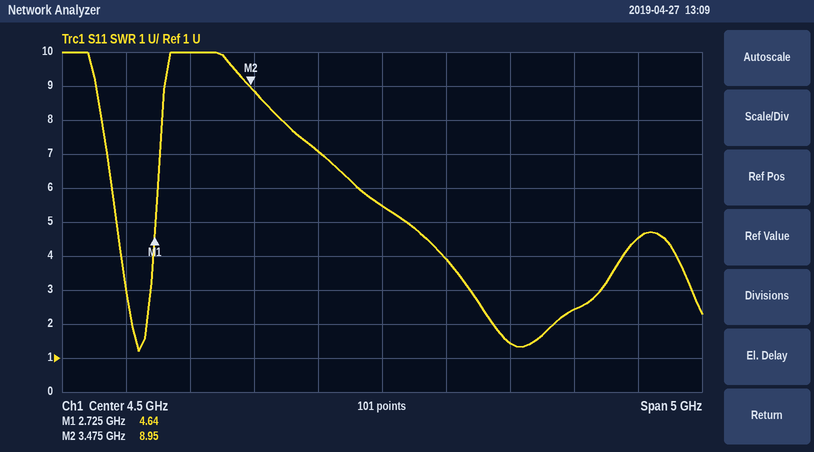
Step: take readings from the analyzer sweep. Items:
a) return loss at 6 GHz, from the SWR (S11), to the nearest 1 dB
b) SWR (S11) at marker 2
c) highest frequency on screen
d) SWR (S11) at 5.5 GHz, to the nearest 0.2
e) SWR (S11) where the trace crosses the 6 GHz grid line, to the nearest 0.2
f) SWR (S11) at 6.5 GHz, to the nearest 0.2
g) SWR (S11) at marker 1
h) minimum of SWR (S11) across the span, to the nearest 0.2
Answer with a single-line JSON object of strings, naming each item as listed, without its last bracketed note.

{"return loss at 6 GHz, from the SWR (S11), to the nearest 1 dB": "8 dB", "SWR (S11) at marker 2": "8.95", "highest frequency on screen": "7 GHz", "SWR (S11) at 5.5 GHz, to the nearest 0.2": "1.4", "SWR (S11) where the trace crosses the 6 GHz grid line, to the nearest 0.2": "2.4", "SWR (S11) at 6.5 GHz, to the nearest 0.2": "4.6", "SWR (S11) at marker 1": "4.64", "minimum of SWR (S11) across the span, to the nearest 0.2": "1.2"}
